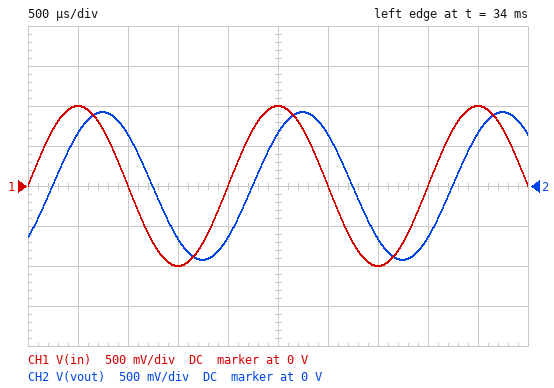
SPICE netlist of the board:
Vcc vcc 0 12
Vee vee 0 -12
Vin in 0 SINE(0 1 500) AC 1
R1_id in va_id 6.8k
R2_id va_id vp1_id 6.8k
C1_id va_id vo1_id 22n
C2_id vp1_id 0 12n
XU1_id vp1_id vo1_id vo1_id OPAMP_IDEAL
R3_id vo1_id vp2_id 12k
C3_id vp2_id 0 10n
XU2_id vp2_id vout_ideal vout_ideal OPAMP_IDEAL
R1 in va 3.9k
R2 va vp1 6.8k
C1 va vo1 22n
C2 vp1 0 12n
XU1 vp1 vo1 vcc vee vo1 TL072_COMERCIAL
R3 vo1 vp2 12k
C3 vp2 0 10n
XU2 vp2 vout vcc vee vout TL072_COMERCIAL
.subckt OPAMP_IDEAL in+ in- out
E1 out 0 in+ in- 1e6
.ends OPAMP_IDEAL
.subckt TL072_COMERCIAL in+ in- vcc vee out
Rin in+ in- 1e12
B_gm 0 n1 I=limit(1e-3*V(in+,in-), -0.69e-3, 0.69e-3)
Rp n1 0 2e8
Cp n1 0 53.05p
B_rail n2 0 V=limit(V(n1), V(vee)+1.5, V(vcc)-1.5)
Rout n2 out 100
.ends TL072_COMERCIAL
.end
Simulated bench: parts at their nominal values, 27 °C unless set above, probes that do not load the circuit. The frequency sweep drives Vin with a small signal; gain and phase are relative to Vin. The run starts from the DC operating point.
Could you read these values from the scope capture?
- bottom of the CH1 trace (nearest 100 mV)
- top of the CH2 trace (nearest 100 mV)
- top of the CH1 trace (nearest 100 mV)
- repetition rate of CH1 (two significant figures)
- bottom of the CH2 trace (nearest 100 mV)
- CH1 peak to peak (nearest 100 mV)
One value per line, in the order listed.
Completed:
-1.0 V
900 mV
1.0 V
500 Hz
-900 mV
2.0 V
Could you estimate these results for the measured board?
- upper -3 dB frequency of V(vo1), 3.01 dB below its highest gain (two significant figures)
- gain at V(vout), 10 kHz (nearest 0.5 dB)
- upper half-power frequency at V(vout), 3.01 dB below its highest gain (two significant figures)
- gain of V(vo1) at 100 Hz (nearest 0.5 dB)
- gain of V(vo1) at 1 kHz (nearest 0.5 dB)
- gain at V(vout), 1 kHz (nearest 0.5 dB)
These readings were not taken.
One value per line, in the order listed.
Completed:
1.7 kHz
-46.5 dB
1.1 kHz
0 dB
-0.5 dB
-2.5 dB
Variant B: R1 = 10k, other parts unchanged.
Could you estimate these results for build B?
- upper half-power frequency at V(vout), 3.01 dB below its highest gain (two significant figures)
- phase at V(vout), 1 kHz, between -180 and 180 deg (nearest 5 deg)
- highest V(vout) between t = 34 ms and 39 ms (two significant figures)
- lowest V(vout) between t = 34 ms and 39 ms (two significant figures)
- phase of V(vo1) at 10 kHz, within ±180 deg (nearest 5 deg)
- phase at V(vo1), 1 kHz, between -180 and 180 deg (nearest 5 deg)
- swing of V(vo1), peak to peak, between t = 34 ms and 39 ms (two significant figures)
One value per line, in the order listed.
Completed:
860 Hz
-115 deg
900 mV
-900 mV
-170 deg
-75 deg
1.9 V
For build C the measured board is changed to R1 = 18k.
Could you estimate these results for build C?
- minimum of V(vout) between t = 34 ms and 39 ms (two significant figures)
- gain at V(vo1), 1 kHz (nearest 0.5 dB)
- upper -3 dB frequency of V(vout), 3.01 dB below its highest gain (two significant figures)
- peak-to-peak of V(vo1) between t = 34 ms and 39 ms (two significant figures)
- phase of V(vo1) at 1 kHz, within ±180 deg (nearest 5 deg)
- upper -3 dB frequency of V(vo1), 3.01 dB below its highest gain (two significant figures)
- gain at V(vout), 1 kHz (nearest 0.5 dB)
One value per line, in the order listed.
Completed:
-810 mV
-5.5 dB
630 Hz
1.7 V
-100 deg
740 Hz
-7.5 dB
